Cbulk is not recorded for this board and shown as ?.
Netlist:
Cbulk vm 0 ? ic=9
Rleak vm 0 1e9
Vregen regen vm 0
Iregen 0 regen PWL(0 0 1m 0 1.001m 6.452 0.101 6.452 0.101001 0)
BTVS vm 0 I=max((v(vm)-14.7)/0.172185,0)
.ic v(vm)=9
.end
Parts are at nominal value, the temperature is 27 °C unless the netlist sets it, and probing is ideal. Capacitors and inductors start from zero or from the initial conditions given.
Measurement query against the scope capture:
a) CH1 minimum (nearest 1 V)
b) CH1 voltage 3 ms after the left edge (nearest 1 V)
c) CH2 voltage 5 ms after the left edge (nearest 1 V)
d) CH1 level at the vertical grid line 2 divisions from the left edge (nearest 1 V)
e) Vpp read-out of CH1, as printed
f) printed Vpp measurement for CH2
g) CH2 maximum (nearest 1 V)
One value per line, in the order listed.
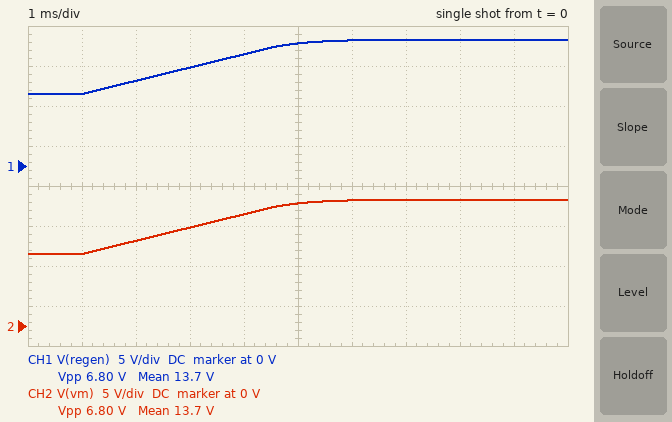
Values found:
9 V
12 V
15 V
11 V
6.80 V
6.80 V
16 V
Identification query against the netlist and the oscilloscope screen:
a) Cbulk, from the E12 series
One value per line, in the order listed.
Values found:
3.9 mF
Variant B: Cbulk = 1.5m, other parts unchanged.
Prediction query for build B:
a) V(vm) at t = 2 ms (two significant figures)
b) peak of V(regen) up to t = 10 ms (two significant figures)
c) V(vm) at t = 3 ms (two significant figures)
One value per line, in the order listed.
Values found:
13 V
16 V
16 V
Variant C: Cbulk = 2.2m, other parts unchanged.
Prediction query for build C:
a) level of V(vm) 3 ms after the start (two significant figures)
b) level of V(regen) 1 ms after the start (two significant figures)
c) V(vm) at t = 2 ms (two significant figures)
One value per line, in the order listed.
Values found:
15 V
9.0 V
12 V
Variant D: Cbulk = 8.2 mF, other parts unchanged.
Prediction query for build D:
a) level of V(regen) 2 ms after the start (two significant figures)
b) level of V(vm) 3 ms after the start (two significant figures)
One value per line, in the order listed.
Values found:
9.8 V
11 V
